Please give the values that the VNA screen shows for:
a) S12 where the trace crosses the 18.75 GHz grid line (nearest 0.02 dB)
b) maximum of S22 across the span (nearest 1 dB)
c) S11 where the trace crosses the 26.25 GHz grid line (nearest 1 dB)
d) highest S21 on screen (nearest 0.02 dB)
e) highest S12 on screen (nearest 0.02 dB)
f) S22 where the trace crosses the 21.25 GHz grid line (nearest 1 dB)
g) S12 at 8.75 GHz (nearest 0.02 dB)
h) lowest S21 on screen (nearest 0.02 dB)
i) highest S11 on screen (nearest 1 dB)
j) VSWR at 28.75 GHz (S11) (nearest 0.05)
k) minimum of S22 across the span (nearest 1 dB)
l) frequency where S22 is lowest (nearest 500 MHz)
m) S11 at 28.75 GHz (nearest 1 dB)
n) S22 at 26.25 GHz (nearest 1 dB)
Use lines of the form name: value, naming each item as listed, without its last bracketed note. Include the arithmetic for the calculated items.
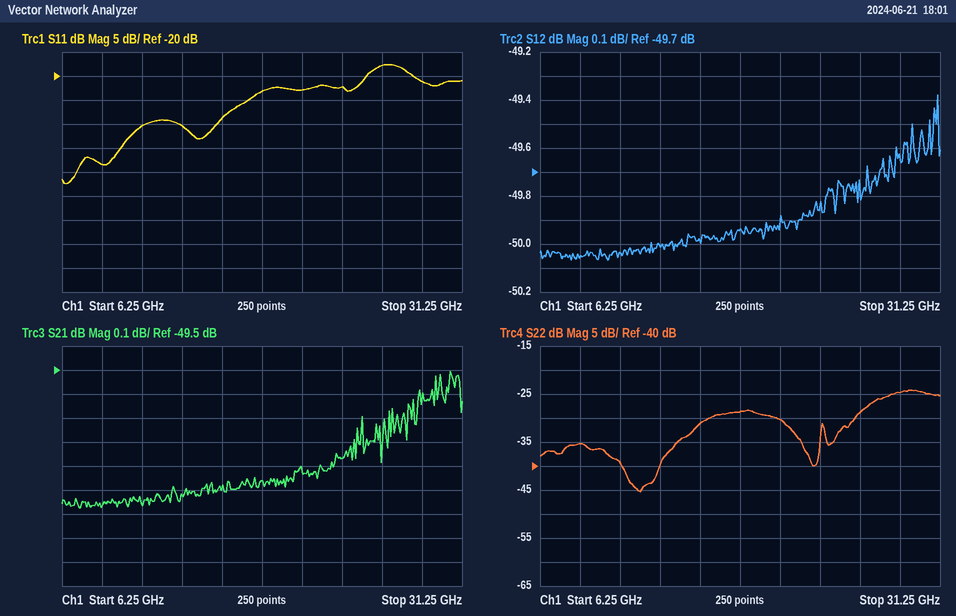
S12 where the trace crosses the 18.75 GHz grid line: -49.94 dB
maximum of S22 across the span: -24 dB
S11 where the trace crosses the 26.25 GHz grid line: -18 dB
highest S21 on screen: -49.50 dB
highest S12 on screen: -49.38 dB
S22 where the trace crosses the 21.25 GHz grid line: -30 dB
S12 at 8.75 GHz: -50.06 dB
lowest S21 on screen: -50.08 dB
highest S11 on screen: -18 dB
VSWR at 28.75 GHz (S11): |Γ| = 10^(-21/20) = 0.0891; VSWR = (1 + 0.0891)/(1 − 0.0891) ≈ 1.20
minimum of S22 across the span: -45 dB
frequency where S22 is lowest: 12.5 GHz
S11 at 28.75 GHz: -21 dB
S22 at 26.25 GHz: -29 dB
